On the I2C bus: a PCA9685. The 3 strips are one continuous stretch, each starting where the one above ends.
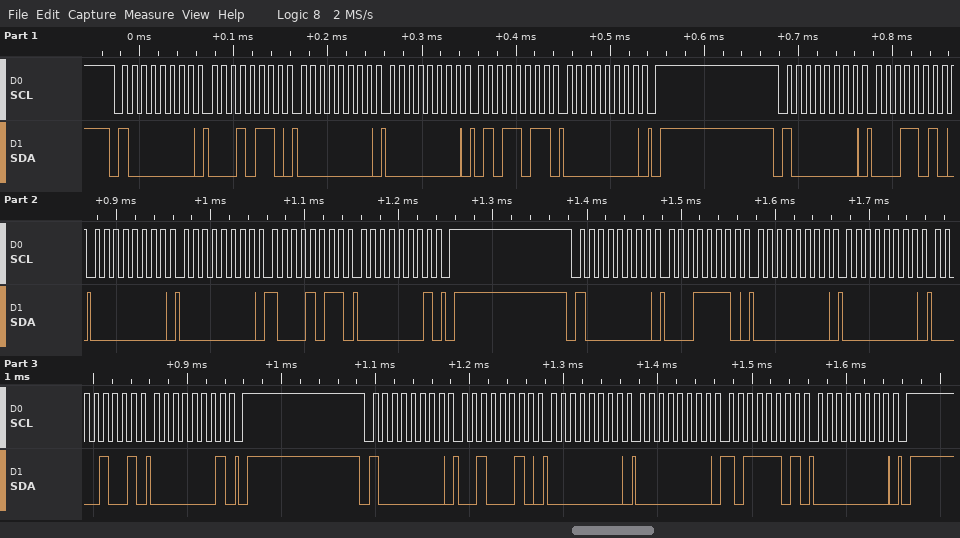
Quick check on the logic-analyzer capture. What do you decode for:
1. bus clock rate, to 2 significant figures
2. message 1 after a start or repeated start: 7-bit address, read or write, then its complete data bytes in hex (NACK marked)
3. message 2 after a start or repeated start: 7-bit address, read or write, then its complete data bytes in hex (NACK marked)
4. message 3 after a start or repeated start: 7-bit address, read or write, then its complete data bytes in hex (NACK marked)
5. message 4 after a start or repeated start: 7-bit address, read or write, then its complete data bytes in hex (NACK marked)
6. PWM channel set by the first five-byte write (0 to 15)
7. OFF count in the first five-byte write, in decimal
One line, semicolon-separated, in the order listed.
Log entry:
100 kHz; 0x40 write: 16 00 00 5B 00; 0x40 write: 1A 00 00 8B 01; 0x40 write: 1E 00 00 09 01; 0x40 write: 22 00 00 BD 00; 4; 91
